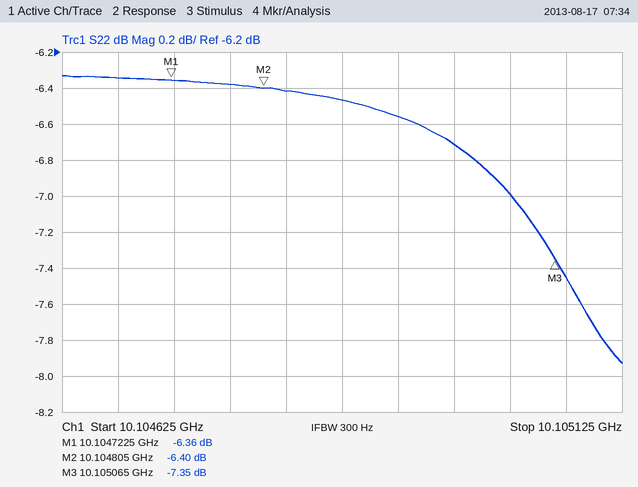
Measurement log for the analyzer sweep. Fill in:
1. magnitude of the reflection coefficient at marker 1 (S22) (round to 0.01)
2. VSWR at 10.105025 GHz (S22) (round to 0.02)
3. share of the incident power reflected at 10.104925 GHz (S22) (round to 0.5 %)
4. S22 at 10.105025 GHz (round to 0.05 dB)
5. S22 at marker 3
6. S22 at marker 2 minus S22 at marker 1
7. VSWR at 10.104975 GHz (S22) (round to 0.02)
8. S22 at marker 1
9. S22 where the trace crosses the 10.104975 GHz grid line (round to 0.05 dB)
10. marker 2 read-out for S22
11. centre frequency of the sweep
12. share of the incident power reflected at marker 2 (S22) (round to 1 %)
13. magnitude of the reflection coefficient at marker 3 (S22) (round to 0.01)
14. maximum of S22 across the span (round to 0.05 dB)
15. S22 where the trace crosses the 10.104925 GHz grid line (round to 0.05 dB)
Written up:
0.48
2.62
22.0 %
-7.00 dB
-7.35 dB
-0.04 dB
2.72
-6.36 dB
-6.70 dB
-6.40 dB
10.104875 GHz
23 %
0.43
-6.35 dB
-6.55 dB
